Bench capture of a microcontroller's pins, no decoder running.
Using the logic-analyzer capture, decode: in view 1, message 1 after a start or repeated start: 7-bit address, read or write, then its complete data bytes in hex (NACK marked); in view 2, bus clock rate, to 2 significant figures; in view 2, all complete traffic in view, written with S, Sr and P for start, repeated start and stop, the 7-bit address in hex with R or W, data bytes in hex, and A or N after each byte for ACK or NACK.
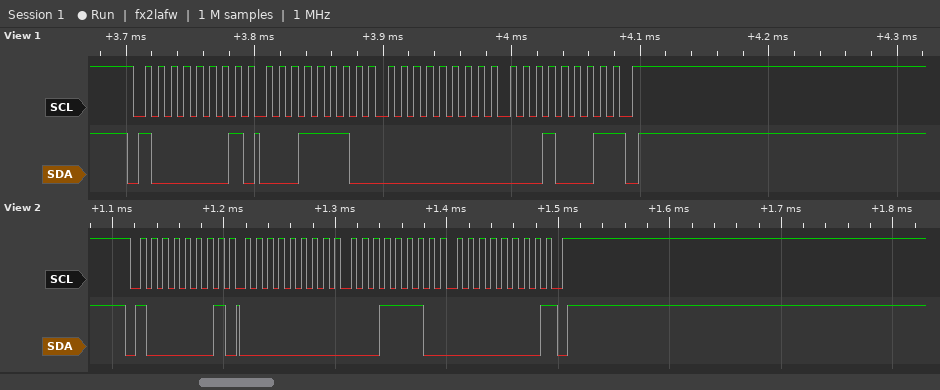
0x40 read: 1E 00 11 NACK
100 kHz
S 40R A 00 A 1E A 00 N P
